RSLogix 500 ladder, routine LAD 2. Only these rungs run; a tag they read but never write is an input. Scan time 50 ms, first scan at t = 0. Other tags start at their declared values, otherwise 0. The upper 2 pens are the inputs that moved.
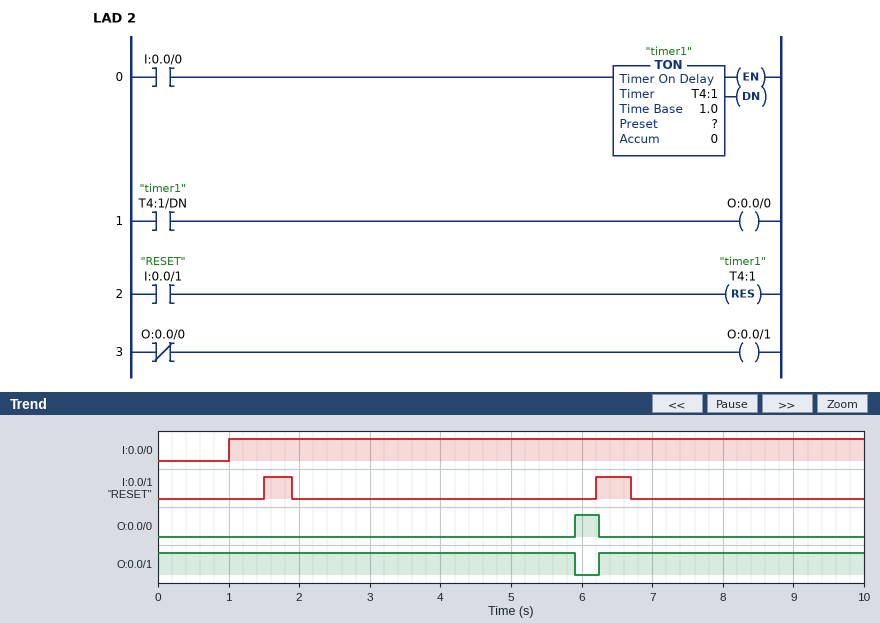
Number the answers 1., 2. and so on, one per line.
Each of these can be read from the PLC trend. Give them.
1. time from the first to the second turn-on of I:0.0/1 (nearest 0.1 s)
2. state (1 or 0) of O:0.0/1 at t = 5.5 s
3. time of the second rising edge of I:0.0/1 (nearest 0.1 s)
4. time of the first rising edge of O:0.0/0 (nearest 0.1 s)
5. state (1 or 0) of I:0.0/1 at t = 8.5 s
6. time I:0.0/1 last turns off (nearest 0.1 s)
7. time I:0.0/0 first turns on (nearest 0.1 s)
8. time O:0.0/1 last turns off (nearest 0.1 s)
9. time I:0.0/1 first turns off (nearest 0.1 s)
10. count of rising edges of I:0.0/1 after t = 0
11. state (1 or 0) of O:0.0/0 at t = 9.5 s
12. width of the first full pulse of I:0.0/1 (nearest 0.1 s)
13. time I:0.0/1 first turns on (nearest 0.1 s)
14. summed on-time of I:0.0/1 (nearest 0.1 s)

1. 4.7 s
2. 1
3. 6.2 s
4. 5.9 s
5. 0
6. 6.7 s
7. 1.0 s
8. 5.9 s
9. 1.9 s
10. 2
11. 0
12. 0.4 s
13. 1.5 s
14. 0.9 s
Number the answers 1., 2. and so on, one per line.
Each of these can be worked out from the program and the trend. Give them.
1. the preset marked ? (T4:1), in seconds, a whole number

1. 4 s
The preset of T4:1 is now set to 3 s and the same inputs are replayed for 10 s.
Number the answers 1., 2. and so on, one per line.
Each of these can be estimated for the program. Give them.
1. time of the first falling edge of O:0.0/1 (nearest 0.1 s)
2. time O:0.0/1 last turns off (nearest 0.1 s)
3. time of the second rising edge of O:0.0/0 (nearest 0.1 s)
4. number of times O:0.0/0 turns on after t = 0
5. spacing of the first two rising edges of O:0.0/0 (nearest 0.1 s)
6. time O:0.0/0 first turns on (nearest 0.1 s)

1. 4.9 s
2. 9.7 s
3. 9.7 s
4. 2
5. 4.8 s
6. 4.9 s
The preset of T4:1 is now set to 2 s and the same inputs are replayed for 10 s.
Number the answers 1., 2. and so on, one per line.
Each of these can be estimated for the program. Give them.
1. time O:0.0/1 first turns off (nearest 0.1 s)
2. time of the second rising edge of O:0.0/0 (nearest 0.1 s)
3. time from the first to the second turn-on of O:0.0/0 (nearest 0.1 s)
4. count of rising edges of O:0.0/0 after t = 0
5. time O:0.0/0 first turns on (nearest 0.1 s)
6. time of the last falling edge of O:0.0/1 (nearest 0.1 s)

1. 3.9 s
2. 8.7 s
3. 4.8 s
4. 2
5. 3.9 s
6. 8.7 s
